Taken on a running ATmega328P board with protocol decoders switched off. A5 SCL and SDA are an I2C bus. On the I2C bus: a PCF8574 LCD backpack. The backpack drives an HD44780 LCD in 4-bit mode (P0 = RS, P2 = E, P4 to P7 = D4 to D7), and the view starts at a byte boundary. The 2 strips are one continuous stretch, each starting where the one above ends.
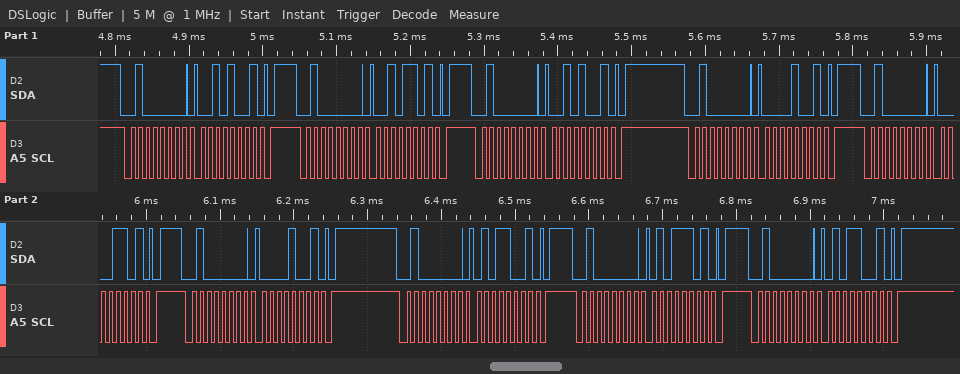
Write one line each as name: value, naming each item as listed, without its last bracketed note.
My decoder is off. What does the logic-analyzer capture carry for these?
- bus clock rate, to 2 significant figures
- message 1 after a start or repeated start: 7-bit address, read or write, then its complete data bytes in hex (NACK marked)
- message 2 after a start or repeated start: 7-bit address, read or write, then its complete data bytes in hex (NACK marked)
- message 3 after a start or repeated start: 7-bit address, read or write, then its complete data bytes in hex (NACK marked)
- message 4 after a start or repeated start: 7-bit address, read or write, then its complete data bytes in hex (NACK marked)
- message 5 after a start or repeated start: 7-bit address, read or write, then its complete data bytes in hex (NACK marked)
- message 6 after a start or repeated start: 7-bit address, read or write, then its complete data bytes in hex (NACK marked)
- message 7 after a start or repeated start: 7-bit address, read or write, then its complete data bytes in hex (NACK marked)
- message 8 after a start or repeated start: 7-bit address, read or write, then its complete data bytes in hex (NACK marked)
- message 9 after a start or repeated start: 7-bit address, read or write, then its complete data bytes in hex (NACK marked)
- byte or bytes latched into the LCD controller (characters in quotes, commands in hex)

bus clock rate, to 2 significant figures: 100 kHz
message 1 after a start or repeated start: 7-bit address, read or write, then its complete data bytes in hex: 0x20 write: 29
message 2 after a start or repeated start: 7-bit address, read or write, then its complete data bytes in hex: 0x20 write: 2D
message 3 after a start or repeated start: 7-bit address, read or write, then its complete data bytes in hex: 0x20 write: 29
message 4 after a start or repeated start: 7-bit address, read or write, then its complete data bytes in hex: 0x20 write: 09
message 5 after a start or repeated start: 7-bit address, read or write, then its complete data bytes in hex: 0x20 write: 0D
message 6 after a start or repeated start: 7-bit address, read or write, then its complete data bytes in hex: 0x20 write: 09
message 7 after a start or repeated start: 7-bit address, read or write, then its complete data bytes in hex: 0x20 write: 59
message 8 after a start or repeated start: 7-bit address, read or write, then its complete data bytes in hex: 0x20 write: 5D
message 9 after a start or repeated start: 7-bit address, read or write, then its complete data bytes in hex: 0x20 write: 59
byte or bytes latched into the LCD controller: ' '
